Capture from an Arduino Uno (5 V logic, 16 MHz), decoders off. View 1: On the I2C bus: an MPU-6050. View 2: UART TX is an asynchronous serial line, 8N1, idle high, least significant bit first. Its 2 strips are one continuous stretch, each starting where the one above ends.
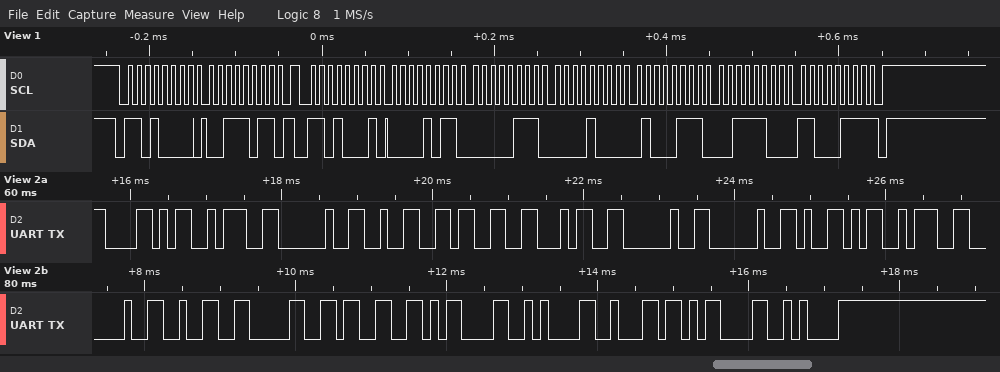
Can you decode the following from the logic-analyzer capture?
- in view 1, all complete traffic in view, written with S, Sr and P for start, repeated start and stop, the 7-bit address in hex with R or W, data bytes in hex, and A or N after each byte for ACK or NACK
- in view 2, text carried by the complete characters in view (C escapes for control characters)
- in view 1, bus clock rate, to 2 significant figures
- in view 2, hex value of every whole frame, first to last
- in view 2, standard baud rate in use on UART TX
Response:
S 68W A 3B A Sr 68R A 0B A 07 A 08 A 47 A 3C A C7 N P
"X: 234  Y: 203\r\nb\r\n"
100 kHz
58 3A 20 32 33 34 20 20 59 3A 20 32 30 33 0D 0A 62 0D 0A
9600 baud
